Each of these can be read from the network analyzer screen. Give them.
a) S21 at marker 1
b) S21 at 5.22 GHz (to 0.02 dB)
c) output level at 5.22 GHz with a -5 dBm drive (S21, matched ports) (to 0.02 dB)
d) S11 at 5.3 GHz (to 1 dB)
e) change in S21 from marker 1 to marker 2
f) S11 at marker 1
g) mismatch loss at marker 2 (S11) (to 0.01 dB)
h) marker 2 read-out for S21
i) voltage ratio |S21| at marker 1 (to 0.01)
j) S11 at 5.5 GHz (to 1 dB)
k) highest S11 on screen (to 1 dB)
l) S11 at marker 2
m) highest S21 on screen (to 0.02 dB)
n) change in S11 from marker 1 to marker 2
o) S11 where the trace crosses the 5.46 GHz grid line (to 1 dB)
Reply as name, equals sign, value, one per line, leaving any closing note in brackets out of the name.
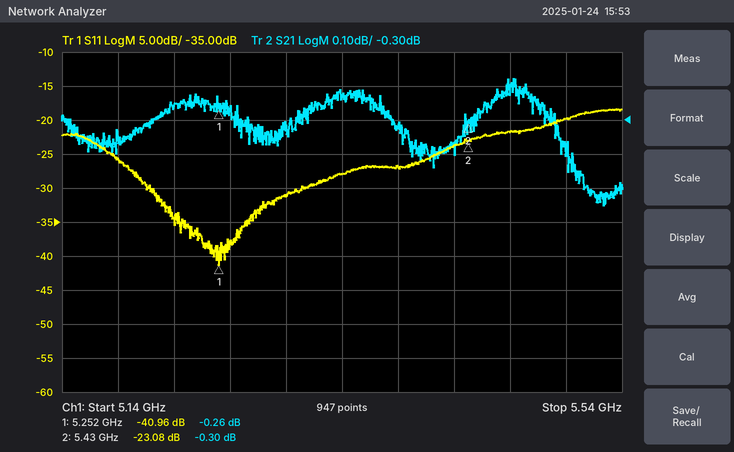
S21 at marker 1 = -0.26 dB
S21 at 5.22 GHz = -0.26 dB
output level at 5.22 GHz with a -5 dBm drive (S21, matched ports) = -5.26 dBm
S11 at 5.3 GHz = -31 dB
change in S21 from marker 1 to marker 2 = -0.04 dB
S11 at marker 1 = -40.96 dB
mismatch loss at marker 2 (S11) = 0.02 dB
marker 2 read-out for S21 = -0.30 dB
voltage ratio |S21| at marker 1 = 0.97
S11 at 5.5 GHz = -20 dB
highest S11 on screen = -18 dB
S11 at marker 2 = -23.08 dB
highest S21 on screen = -0.18 dB
change in S11 from marker 1 to marker 2 = 17.88 dB
S11 where the trace crosses the 5.46 GHz grid line = -22 dB
